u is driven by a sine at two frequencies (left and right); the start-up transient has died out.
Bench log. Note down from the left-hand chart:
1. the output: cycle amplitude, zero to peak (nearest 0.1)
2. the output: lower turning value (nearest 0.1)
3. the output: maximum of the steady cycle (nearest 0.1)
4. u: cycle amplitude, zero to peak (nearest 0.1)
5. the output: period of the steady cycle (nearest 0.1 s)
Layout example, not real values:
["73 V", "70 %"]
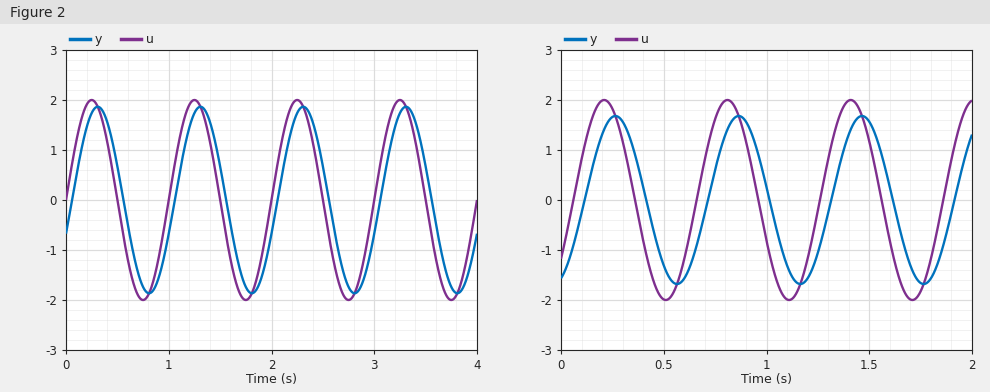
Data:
["1.9", "-1.9", "1.9", "2.0", "1.0 s"]
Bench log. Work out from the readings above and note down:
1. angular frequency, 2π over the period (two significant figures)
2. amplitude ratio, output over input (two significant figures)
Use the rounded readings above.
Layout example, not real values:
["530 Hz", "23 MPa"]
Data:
["6.3 rad/s", "0.95"]
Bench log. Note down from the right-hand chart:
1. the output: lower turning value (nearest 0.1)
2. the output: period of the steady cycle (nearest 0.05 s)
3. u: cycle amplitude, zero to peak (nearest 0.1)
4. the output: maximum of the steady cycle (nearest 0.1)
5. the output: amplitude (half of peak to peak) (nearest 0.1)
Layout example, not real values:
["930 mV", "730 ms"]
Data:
["-1.7", "0.60 s", "2.0", "1.7", "1.7"]
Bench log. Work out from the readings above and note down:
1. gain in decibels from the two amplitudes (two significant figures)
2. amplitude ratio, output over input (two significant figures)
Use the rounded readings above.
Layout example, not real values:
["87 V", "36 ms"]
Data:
["-1.4 dB", "0.85"]
